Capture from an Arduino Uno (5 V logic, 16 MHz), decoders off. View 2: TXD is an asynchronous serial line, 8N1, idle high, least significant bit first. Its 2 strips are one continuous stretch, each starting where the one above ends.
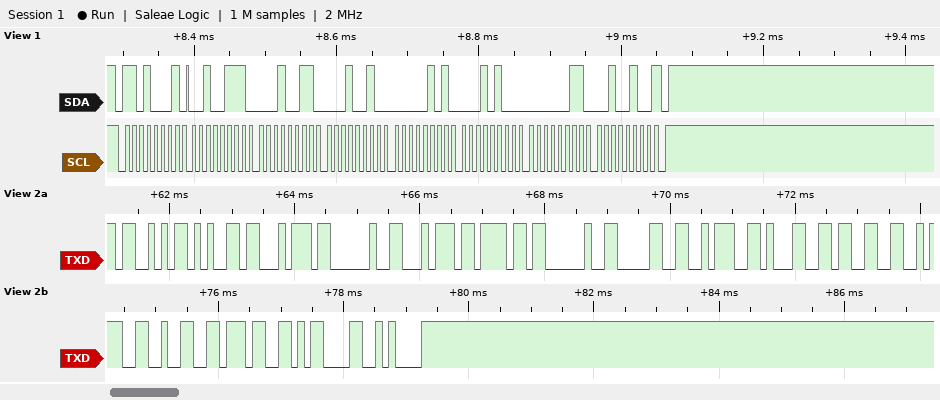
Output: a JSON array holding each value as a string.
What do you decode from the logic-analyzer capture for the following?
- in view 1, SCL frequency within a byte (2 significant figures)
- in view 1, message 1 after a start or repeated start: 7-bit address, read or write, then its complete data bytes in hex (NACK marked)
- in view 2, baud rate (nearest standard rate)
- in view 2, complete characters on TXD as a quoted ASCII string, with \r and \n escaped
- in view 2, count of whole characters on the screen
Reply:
["100 kHz", "0x68 read: 27 13 12 05 14 03 24 NACK", "9600 baud", "\"Set to 0:13:27\\r\\n\"", "16"]
